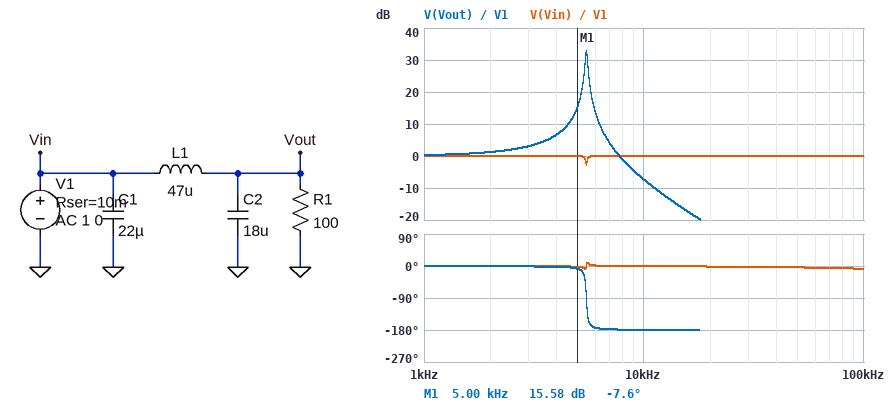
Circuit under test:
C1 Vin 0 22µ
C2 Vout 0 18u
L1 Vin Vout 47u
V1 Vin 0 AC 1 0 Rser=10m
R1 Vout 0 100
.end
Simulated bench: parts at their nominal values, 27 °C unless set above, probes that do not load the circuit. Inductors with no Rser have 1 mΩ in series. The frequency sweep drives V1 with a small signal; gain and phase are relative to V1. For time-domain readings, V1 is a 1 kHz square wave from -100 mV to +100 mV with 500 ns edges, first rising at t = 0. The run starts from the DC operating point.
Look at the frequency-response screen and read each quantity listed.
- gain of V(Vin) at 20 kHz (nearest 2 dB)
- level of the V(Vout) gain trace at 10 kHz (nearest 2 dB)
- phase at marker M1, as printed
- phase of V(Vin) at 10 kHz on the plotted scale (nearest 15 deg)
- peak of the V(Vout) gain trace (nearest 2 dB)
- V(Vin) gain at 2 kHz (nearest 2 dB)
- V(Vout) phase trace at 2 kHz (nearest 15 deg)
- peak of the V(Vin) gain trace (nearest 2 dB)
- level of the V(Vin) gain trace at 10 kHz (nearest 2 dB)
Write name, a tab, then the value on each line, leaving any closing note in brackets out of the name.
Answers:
gain of V(Vin) at 20 kHz	0 dB
level of the V(Vout) gain trace at 10 kHz	-8 dB
phase at marker M1, as printed	-7.6 deg
phase of V(Vin) at 10 kHz on the plotted scale	0 deg
peak of the V(Vout) gain trace	32 dB
V(Vin) gain at 2 kHz	0 dB
V(Vout) phase trace at 2 kHz	0 deg
peak of the V(Vin) gain trace	0 dB
level of the V(Vin) gain trace at 10 kHz	0 dB
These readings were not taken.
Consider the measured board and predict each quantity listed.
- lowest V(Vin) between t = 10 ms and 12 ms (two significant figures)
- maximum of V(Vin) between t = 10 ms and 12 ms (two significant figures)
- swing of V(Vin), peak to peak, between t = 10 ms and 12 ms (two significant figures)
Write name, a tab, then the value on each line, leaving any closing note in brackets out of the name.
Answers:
lowest V(Vin) between t = 10 ms and 12 ms	-100 mV
maximum of V(Vin) between t = 10 ms and 12 ms	100 mV
swing of V(Vin), peak to peak, between t = 10 ms and 12 ms	200 mV
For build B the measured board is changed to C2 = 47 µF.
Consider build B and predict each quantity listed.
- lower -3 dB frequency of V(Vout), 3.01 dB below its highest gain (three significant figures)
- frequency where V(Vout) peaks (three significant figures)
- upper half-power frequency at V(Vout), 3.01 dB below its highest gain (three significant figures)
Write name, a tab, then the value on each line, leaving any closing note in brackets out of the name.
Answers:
lower -3 dB frequency of V(Vout), 3.01 dB below its highest gain	3.35 kHz
frequency where V(Vout) peaks	3.39 kHz
upper half-power frequency at V(Vout), 3.01 dB below its highest gain	3.42 kHz
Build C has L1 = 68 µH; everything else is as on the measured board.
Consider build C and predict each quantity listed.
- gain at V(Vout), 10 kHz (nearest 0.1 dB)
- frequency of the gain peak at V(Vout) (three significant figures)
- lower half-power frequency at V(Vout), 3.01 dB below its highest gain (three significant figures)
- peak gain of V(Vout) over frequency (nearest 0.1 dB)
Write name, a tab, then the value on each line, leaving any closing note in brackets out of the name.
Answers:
gain at V(Vout), 10 kHz	-11.7 dB
frequency of the gain peak at V(Vout)	4.55 kHz
lower half-power frequency at V(Vout), 3.01 dB below its highest gain	4.49 kHz
peak gain of V(Vout) over frequency	32.0 dB
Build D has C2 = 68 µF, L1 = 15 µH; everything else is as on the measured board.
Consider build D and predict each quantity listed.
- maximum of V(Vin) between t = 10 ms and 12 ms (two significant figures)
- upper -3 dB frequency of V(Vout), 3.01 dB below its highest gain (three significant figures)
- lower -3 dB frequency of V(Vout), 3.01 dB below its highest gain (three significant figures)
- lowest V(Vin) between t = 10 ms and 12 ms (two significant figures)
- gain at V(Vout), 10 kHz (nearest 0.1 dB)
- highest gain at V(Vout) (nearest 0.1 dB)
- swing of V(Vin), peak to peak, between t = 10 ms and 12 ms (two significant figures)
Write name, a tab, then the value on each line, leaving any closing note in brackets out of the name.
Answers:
maximum of V(Vin) between t = 10 ms and 12 ms	120 mV
upper -3 dB frequency of V(Vout), 3.01 dB below its highest gain	5.05 kHz
lower -3 dB frequency of V(Vout), 3.01 dB below its highest gain	4.91 kHz
lowest V(Vin) between t = 10 ms and 12 ms	-120 mV
gain at V(Vout), 10 kHz	-9.6 dB
highest gain at V(Vout)	31.0 dB
swing of V(Vin), peak to peak, between t = 10 ms and 12 ms	240 mV
